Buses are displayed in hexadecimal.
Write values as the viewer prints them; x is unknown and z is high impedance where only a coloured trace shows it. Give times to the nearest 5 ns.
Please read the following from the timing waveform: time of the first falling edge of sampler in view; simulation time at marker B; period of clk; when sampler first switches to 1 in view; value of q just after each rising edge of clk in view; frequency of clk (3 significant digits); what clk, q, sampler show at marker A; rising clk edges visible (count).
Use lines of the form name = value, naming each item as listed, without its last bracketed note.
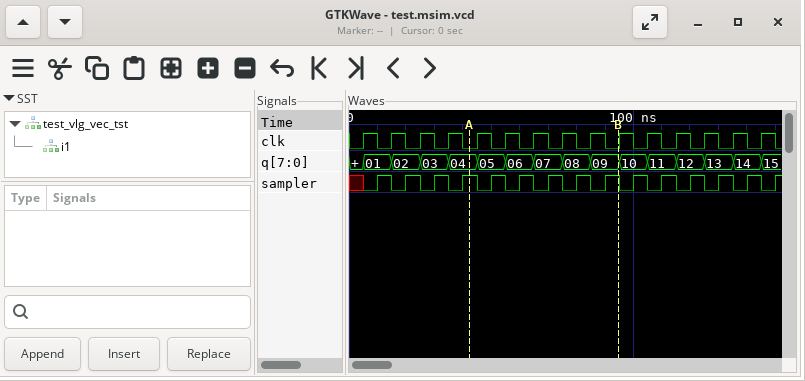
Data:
time of the first falling edge of sampler in view = 15 ns
simulation time at marker B = 95 ns
period of clk = 10 ns
when sampler first switches to 1 in view = 10 ns
value of q just after each rising edge of clk in view = 01, 02, 03, 04, 05, 06, 07, 08, 09, 10, 11, 12, 13, 14, 15
frequency of clk = 100 MHz
what clk, q, sampler show at marker A = clk=0, q=04, sampler=1
rising clk edges visible = 15
